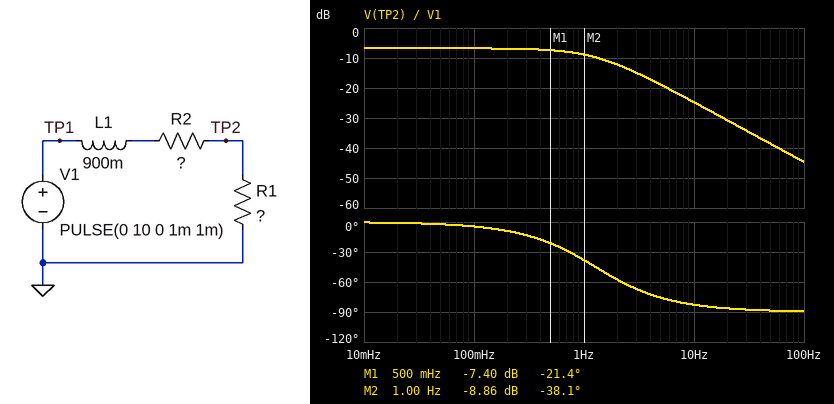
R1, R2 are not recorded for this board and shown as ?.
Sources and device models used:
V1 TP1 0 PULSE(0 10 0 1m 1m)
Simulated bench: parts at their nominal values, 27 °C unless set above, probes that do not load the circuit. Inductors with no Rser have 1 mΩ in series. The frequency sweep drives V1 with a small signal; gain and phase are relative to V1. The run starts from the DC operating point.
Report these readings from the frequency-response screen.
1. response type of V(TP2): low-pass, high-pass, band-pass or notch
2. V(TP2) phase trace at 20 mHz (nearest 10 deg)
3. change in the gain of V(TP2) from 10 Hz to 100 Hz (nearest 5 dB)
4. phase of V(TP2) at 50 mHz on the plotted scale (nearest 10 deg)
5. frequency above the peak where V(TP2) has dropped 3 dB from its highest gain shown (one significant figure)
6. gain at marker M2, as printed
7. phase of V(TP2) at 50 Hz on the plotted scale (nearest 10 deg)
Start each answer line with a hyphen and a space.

- low-pass
- 0 deg
- -20 dB
- 0 deg
- 1 Hz
- -8.86 dB
- -90 deg
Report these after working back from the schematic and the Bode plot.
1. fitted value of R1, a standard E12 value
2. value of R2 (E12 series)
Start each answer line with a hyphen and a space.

- 3.3 Ω
- 3.9 Ω
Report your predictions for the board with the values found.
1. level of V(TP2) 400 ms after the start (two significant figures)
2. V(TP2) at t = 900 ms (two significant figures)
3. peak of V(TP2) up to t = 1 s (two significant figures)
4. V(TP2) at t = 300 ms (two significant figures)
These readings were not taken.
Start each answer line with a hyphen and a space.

- 4.4 V
- 4.6 V
- 4.6 V
- 4.2 V
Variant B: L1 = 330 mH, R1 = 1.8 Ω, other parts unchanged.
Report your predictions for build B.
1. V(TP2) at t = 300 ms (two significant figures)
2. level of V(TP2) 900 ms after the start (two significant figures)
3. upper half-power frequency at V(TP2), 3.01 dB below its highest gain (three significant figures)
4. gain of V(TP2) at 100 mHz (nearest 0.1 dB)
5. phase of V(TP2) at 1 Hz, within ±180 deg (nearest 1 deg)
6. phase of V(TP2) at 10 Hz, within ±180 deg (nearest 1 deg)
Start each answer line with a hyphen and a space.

- 3.1 V
- 3.2 V
- 2.75 Hz
- -10.0 dB
- -20 deg
- -75 deg
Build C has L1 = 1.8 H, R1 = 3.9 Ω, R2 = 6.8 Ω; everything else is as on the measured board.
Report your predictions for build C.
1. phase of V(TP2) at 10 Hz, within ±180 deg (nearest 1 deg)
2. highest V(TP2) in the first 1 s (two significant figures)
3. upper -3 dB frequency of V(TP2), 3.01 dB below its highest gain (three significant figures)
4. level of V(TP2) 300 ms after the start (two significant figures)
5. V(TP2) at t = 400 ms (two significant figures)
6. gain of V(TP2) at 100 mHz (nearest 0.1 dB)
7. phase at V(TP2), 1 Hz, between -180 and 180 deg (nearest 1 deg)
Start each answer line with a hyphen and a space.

- -85 deg
- 3.6 V
- 946 mHz
- 3.0 V
- 3.3 V
- -8.8 dB
- -47 deg
